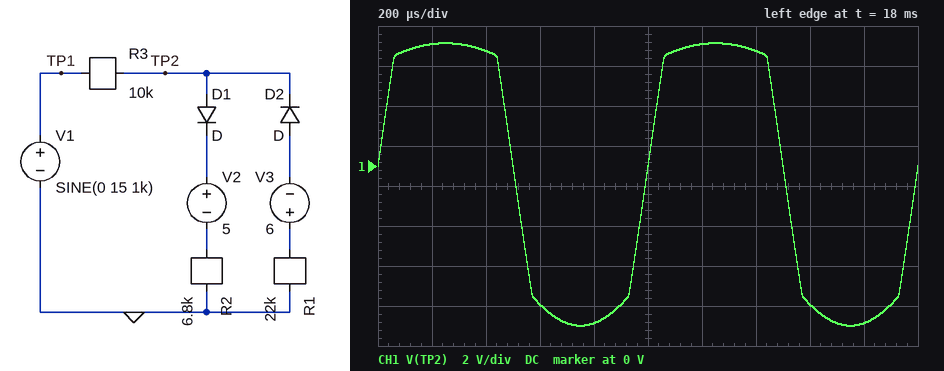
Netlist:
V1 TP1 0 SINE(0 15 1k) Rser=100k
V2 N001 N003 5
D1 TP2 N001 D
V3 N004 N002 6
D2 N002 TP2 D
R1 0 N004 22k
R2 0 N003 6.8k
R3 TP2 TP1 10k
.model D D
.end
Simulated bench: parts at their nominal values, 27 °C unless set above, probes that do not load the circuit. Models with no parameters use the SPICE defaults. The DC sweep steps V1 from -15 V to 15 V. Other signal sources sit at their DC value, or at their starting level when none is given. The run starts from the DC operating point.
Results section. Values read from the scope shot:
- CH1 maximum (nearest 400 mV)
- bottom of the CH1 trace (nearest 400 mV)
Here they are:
6.0 V
-8.0 V
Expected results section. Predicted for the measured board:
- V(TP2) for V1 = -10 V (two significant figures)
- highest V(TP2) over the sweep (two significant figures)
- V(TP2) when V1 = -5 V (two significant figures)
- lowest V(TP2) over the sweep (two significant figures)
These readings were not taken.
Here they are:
-7.1 V
6.1 V
-5.0 V
-8.0 V
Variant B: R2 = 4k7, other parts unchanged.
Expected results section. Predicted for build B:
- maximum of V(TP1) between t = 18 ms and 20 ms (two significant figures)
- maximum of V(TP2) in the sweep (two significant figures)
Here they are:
6.8 V
6.0 V
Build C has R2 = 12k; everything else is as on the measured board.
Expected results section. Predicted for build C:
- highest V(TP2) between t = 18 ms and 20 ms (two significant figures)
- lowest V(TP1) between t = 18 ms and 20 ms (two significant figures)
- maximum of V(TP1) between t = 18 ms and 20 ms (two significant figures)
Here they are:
6.5 V
-8.6 V
7.3 V
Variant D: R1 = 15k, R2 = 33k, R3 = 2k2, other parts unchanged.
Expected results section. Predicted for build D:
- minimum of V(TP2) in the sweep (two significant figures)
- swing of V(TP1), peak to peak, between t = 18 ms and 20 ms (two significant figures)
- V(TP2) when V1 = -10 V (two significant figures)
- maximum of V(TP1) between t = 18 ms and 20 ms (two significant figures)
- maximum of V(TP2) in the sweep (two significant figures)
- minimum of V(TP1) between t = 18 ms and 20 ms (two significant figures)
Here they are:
-7.7 V
16 V
-7.0 V
8.0 V
7.9 V
-7.8 V
